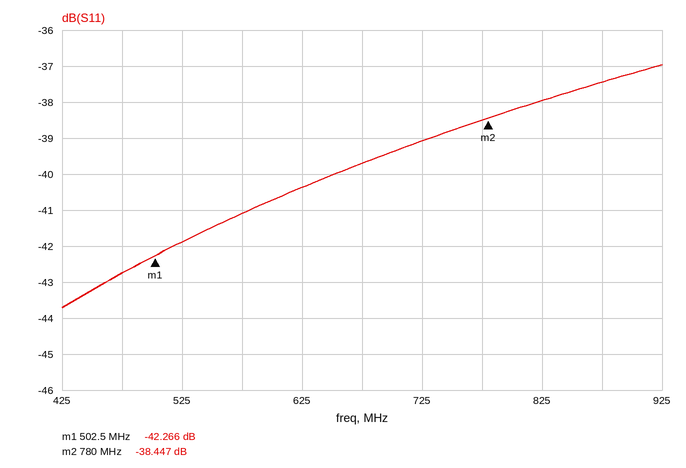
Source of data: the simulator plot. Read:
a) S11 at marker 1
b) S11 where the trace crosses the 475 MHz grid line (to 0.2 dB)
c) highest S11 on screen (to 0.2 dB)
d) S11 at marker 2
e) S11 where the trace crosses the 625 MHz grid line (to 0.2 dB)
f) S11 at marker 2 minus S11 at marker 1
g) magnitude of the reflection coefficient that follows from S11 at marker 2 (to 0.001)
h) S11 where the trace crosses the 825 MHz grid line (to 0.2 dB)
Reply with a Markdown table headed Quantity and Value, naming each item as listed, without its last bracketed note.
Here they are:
| Quantity | Value |
|---|---|
| S11 at marker 1 | -42.266 dB |
| S11 where the trace crosses the 475 MHz grid line | -42.8 dB |
| highest S11 on screen | -37.0 dB |
| S11 at marker 2 | -38.447 dB |
| S11 where the trace crosses the 625 MHz grid line | -40.4 dB |
| S11 at marker 2 minus S11 at marker 1 | 3.819 dB |
| magnitude of the reflection coefficient that follows from S11 at marker 2 | 0.012 |
| S11 where the trace crosses the 825 MHz grid line | -38.0 dB |
